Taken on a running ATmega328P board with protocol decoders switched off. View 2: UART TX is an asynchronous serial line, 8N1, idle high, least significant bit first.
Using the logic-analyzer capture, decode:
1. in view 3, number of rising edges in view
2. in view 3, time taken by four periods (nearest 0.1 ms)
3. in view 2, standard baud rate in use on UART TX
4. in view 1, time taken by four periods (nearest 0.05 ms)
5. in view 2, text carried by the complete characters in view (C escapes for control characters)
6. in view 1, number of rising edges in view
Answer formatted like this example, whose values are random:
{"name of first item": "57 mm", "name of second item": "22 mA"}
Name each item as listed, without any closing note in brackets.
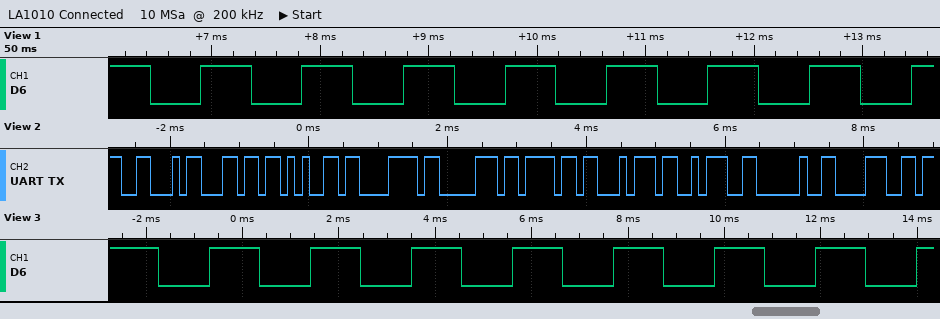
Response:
{"in view 3, number of rising edges in view": "8", "in view 3, time taken by four periods": "8.4 ms", "in view 2, standard baud rate in use on UART TX": "9600 baud", "in view 1, time taken by four periods": "3.75 ms", "in view 2, text carried by the complete characters in view": "\"Flexpot: 8\"", "in view 1, number of rising edges in view": "8"}
